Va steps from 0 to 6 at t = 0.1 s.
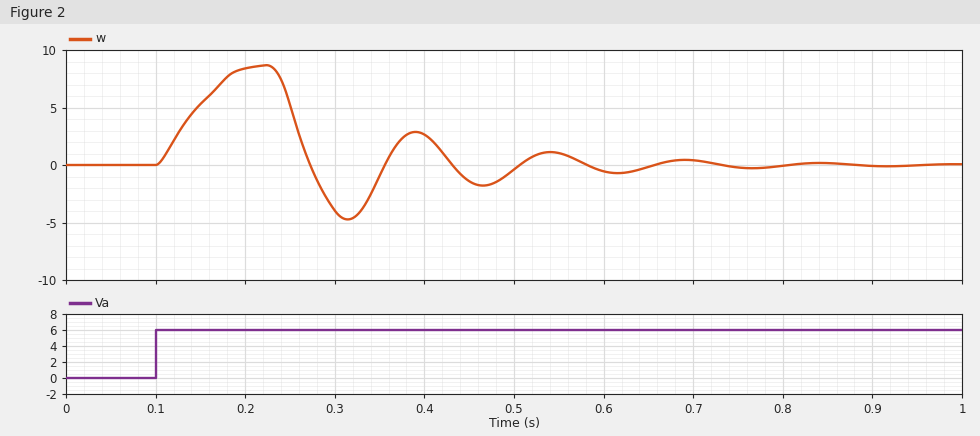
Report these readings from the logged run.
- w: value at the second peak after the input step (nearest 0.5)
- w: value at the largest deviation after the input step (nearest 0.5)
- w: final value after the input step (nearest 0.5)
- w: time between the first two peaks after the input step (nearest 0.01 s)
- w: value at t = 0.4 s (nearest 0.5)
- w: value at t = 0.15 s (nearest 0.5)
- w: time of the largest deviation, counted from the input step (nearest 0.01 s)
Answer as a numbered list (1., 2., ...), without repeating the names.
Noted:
1. 3.0
2. 8.5
3. 0.0
4. 0.17 s
5. 2.5
6. 5.5
7. 0.12 s
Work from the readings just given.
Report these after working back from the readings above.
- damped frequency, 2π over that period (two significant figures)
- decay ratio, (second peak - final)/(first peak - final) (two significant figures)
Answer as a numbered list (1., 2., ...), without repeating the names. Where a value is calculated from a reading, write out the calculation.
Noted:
1. 2π / 0.17 = 37 rad/s
2. (3 - 0) / (8.5 - 0) = 0.35
